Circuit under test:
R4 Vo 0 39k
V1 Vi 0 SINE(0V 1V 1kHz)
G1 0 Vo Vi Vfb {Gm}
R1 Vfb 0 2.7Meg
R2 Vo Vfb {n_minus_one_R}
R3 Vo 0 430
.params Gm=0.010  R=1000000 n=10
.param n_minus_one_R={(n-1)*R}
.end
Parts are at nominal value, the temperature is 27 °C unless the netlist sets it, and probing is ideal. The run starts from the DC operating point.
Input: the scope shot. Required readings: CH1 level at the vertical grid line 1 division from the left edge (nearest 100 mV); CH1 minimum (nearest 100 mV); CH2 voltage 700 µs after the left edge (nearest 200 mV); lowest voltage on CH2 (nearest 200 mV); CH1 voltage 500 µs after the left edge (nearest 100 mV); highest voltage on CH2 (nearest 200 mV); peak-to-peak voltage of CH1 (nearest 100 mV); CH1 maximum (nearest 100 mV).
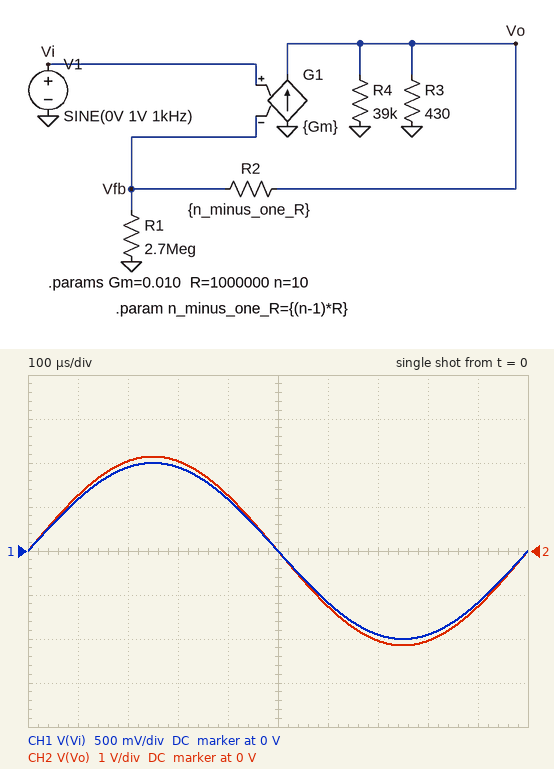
600 mV
-1.0 V
-2.0 V
-2.2 V
0 V
2.2 V
2.0 V
1.0 V
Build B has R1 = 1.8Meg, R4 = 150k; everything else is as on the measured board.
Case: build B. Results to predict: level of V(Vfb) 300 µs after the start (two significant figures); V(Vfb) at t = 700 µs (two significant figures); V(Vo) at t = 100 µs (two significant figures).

400 mV
-400 mV
1.5 V
